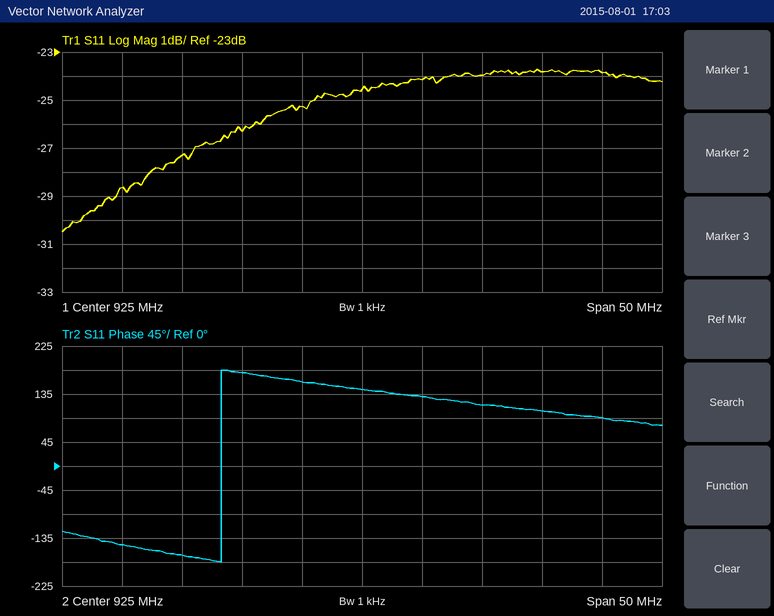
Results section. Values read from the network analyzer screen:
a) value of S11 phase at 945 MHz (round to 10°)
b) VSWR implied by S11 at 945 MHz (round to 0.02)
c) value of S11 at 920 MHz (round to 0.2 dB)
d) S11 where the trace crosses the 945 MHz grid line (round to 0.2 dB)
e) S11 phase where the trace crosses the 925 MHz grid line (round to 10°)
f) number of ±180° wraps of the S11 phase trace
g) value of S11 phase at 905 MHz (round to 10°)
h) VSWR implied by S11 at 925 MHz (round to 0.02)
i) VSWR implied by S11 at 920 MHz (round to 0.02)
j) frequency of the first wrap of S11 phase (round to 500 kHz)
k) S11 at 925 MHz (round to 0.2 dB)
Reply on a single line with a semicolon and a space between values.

90°; 1.14; -25.2 dB; -23.8 dB; 140°; 1; -150°; 1.12; 1.12; 913.5 MHz; -24.6 dB
